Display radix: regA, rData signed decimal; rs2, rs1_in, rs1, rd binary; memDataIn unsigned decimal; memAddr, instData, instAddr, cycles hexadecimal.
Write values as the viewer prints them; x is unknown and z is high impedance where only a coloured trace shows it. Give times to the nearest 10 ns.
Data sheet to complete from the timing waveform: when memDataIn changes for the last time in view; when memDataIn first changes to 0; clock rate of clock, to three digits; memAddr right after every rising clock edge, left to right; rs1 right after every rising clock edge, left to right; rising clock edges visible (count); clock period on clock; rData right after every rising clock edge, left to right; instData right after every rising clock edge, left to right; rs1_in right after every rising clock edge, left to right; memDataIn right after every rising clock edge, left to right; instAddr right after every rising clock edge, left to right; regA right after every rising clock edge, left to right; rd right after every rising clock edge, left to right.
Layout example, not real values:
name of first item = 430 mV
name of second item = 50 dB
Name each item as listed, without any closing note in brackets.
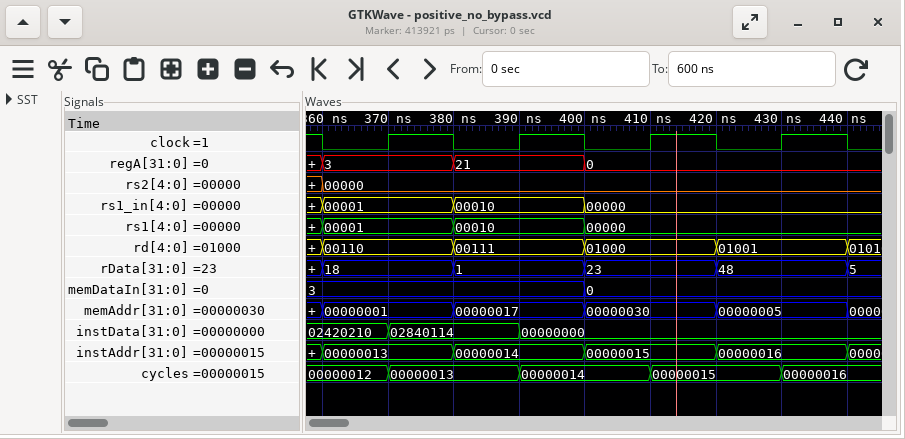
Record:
when memDataIn changes for the last time in view = 400 ns
when memDataIn first changes to 0 = 400 ns
clock rate of clock, to three digits = 50.0 MHz
memAddr right after every rising clock edge, left to right = 00000001, 00000017, 00000030, 00000005
rs1 right after every rising clock edge, left to right = 00001, 00010, 00000, 00000
rising clock edges visible = 4
clock period on clock = 20 ns
rData right after every rising clock edge, left to right = 18, 1, 23, 48
instData right after every rising clock edge, left to right = 02840114, 00000000, 00000000, 00000000
rs1_in right after every rising clock edge, left to right = 00001, 00010, 00000, 00000
memDataIn right after every rising clock edge, left to right = 3, 3, 0, 0
instAddr right after every rising clock edge, left to right = 00000013, 00000014, 00000015, 00000016
regA right after every rising clock edge, left to right = 3, 21, 0, 0
rd right after every rising clock edge, left to right = 00110, 00111, 01000, 01001
